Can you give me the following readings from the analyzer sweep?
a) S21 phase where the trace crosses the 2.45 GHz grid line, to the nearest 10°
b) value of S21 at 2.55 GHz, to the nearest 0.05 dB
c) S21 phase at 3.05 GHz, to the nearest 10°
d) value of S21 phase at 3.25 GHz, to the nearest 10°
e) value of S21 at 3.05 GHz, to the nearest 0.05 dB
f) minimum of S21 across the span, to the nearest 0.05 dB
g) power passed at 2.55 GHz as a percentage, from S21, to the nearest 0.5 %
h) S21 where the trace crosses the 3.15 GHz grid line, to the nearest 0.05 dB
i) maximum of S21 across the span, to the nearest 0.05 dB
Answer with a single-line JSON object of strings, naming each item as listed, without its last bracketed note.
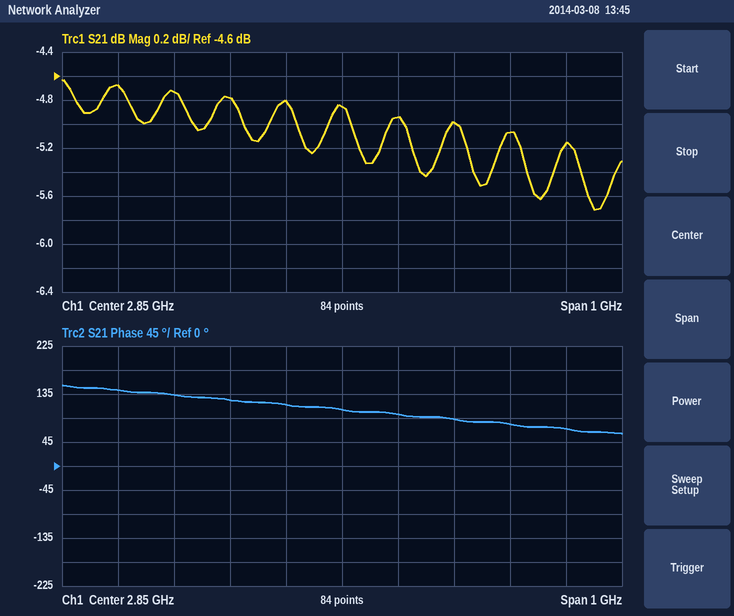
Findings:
{"S21 phase where the trace crosses the 2.45 GHz grid line, to the nearest 10°": "140°", "value of S21 at 2.55 GHz, to the nearest 0.05 dB": "-4.75 dB", "S21 phase at 3.05 GHz, to the nearest 10°": "90°", "value of S21 phase at 3.25 GHz, to the nearest 10°": "70°", "value of S21 at 3.05 GHz, to the nearest 0.05 dB": "-5.00 dB", "minimum of S21 across the span, to the nearest 0.05 dB": "-5.70 dB", "power passed at 2.55 GHz as a percentage, from S21, to the nearest 0.5 %": "33.5 %", "S21 where the trace crosses the 3.15 GHz grid line, to the nearest 0.05 dB": "-5.05 dB", "maximum of S21 across the span, to the nearest 0.05 dB": "-4.65 dB"}
